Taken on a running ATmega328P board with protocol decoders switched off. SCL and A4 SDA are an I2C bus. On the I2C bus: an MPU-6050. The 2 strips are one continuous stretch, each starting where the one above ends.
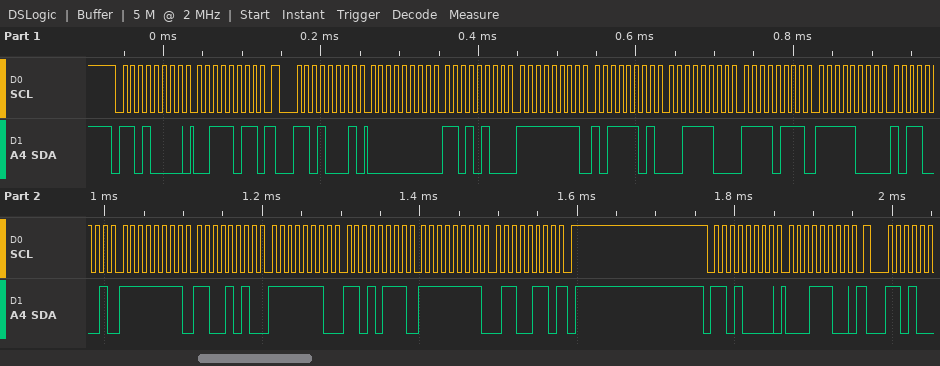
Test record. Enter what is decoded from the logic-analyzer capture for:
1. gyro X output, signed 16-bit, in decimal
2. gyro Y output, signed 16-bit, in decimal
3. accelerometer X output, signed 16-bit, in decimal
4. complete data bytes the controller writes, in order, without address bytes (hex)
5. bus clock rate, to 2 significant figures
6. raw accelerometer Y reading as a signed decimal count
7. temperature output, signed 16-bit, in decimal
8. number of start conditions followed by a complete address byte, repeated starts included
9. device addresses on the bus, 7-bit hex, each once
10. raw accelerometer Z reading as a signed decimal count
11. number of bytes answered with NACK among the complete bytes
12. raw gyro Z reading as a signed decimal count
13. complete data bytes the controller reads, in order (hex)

-54
-297
212
3B 1C
100 kHz
-67
-1871
3
0x68
15607
1
-154
00 D4 FF BD 3C F7 F8 B1 FF CA FE D7 FF 66
